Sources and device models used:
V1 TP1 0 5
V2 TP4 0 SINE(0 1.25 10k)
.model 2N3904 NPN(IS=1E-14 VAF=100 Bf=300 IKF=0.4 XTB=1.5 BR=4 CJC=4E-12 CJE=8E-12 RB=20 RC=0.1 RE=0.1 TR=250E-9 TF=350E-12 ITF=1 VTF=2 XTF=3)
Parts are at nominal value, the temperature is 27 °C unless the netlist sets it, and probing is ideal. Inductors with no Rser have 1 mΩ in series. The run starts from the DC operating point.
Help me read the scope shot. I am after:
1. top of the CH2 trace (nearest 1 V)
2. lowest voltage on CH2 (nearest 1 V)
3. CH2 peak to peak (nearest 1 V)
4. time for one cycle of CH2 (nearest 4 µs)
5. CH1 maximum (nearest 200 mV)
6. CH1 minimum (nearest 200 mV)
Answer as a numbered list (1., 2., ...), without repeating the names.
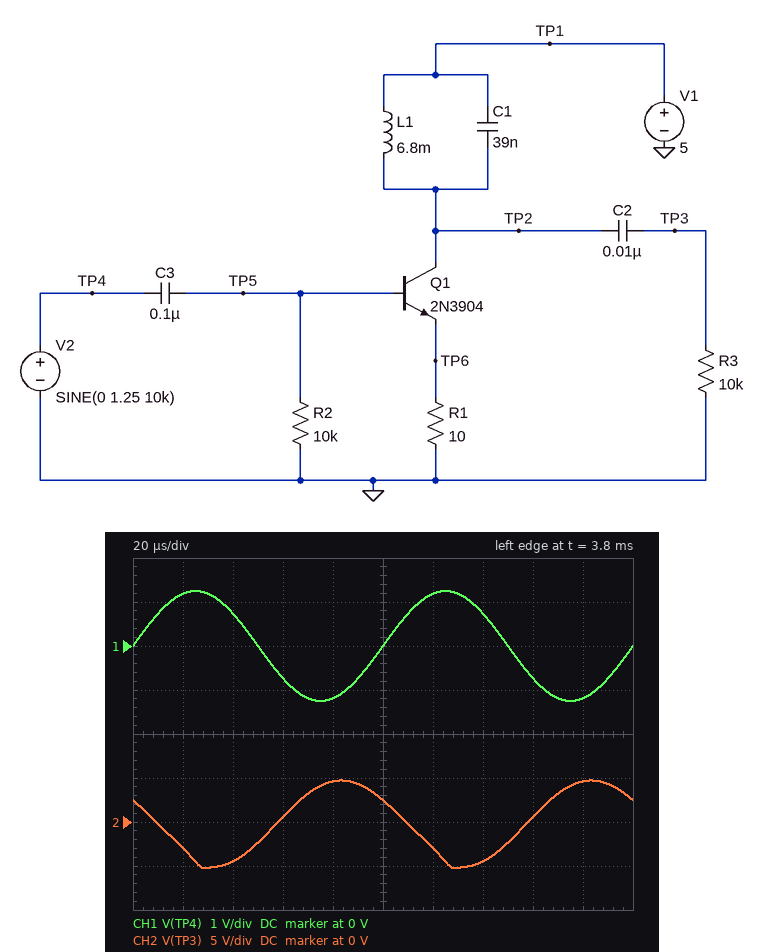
1. 5 V
2. -5 V
3. 10 V
4. 100 µs
5. 1.2 V
6. -1.2 V
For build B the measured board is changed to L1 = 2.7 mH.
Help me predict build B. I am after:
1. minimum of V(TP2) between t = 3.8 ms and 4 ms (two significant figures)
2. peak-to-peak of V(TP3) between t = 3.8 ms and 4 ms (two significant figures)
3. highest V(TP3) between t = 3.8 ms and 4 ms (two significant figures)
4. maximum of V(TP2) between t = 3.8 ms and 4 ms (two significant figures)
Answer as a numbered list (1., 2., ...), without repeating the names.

1. -750 mV
2. 12 V
3. 5.8 V
4. 11 V
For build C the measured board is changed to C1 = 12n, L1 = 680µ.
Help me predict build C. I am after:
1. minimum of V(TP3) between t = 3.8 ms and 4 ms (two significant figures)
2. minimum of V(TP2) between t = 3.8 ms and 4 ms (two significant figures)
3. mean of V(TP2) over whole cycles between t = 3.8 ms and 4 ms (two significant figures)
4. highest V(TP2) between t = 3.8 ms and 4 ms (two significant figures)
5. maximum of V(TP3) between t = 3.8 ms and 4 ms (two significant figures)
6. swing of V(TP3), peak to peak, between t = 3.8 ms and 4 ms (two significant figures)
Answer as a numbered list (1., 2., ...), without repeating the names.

1. -4.3 V
2. 560 mV
3. 5.0 V
4. 9.3 V
5. 4.4 V
6. 8.7 V
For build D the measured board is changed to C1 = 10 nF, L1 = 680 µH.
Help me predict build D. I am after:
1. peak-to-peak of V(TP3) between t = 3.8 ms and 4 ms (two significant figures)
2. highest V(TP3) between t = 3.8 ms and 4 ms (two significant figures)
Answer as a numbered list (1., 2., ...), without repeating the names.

1. 6.0 V
2. 2.6 V
